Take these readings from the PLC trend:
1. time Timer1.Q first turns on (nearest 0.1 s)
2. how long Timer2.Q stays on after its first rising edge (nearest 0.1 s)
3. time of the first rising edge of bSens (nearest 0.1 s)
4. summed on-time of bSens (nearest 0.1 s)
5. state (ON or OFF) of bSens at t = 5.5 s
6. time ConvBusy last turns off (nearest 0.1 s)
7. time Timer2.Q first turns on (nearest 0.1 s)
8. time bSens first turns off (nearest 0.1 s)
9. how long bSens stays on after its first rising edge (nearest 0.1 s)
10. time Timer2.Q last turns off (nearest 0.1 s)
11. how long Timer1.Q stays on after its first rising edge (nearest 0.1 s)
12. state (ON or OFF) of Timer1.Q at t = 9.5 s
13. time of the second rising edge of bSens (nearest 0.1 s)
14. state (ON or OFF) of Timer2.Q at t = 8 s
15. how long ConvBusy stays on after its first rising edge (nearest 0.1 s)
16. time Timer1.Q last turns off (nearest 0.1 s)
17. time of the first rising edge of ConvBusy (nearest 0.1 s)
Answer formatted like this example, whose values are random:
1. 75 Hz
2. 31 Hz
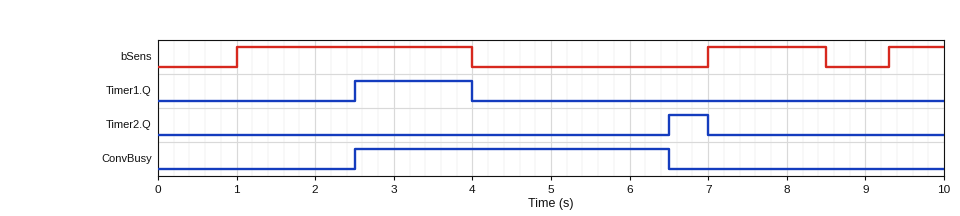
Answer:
1. 2.5 s
2. 0.5 s
3. 1.0 s
4. 5.2 s
5. OFF
6. 6.5 s
7. 6.5 s
8. 4.0 s
9. 3.0 s
10. 7.0 s
11. 1.5 s
12. OFF
13. 7.0 s
14. OFF
15. 4.0 s
16. 4.0 s
17. 2.5 s
